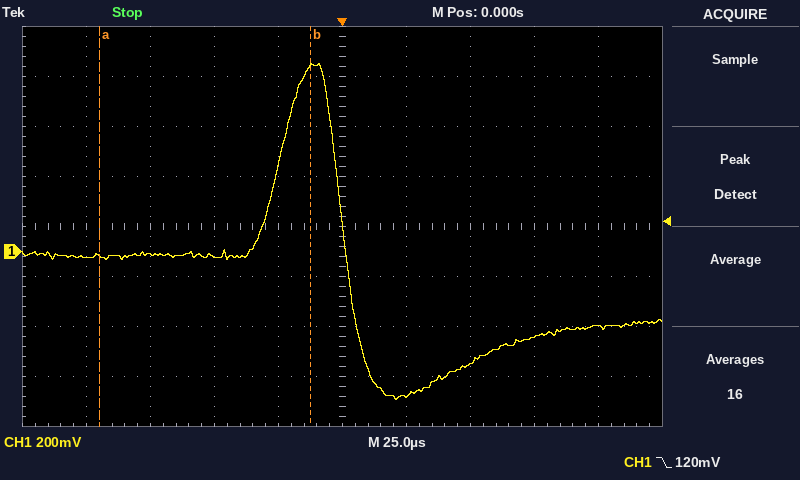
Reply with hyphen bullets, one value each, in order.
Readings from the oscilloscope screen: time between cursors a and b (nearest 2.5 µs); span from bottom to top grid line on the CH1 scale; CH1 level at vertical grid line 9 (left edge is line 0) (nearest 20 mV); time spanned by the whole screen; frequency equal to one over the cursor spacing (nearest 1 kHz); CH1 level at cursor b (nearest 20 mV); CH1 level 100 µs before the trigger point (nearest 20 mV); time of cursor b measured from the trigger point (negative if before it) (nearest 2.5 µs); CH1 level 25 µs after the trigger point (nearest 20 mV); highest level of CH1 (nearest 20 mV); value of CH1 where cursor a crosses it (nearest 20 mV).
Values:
- 82.5 µs
- 1.6 V
- -300 mV
- 250 µs
- 12 kHz
- 740 mV
- -20 mV
- -12.5 µs
- -580 mV
- 760 mV
- -20 mV
